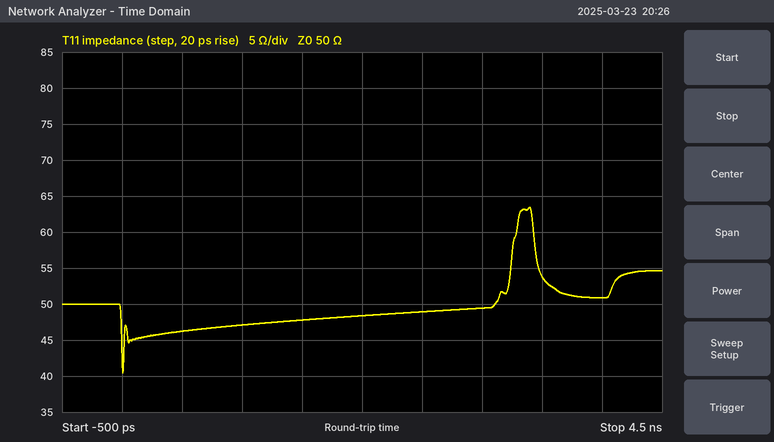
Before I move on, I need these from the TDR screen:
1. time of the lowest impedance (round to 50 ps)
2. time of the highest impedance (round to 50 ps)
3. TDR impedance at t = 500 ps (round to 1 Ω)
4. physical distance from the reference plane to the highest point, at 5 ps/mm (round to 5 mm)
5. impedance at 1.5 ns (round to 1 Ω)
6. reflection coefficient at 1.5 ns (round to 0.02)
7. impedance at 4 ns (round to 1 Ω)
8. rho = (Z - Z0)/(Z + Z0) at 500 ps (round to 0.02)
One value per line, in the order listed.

0 ps
3.40 ns
46 Ω
340 mm
48 Ω
-0.02
51 Ω
-0.04
